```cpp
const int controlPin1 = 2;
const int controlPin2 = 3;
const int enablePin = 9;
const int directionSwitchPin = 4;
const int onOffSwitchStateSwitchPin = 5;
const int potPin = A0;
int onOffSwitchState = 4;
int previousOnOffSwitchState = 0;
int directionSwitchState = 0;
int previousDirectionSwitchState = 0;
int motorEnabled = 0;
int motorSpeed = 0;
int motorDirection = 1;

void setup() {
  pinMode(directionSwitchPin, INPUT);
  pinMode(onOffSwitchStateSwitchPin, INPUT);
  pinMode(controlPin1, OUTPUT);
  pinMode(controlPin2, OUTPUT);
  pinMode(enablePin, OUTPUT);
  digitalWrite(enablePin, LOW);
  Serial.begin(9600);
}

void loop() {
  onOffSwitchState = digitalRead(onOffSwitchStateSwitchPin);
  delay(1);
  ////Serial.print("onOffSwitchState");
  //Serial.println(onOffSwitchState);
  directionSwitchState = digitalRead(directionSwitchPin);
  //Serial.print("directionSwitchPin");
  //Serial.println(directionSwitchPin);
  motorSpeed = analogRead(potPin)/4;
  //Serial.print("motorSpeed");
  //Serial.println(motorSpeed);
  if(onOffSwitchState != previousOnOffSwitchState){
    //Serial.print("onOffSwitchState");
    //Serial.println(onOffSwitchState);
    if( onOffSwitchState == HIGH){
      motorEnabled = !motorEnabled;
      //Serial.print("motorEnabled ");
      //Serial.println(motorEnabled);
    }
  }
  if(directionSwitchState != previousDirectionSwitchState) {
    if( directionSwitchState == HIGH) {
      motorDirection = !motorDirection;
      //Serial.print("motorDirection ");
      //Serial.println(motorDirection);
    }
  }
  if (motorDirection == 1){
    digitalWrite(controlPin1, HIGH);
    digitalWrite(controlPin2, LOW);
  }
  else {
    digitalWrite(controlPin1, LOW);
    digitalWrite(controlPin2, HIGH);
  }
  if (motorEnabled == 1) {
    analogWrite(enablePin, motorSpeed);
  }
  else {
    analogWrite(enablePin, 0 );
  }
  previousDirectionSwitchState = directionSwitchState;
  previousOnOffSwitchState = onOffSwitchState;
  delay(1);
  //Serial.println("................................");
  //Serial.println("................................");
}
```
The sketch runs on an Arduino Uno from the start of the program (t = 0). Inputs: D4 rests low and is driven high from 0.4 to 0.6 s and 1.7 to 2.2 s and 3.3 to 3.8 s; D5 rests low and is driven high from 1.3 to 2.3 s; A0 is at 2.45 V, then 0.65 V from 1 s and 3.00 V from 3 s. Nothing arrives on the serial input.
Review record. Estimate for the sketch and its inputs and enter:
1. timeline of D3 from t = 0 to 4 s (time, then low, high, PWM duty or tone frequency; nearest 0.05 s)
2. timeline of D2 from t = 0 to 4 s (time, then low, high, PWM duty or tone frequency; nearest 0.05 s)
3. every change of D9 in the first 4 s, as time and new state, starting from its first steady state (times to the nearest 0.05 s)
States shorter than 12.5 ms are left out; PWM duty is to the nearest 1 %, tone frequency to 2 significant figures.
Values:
0 s low; 0.4 s high; 1.7 s low; 3.3 s high
0 s high; 0.4 s low; 1.7 s high; 3.3 s low
0 s low; 1.3 s PWM 13 %; 3 s PWM 60 %
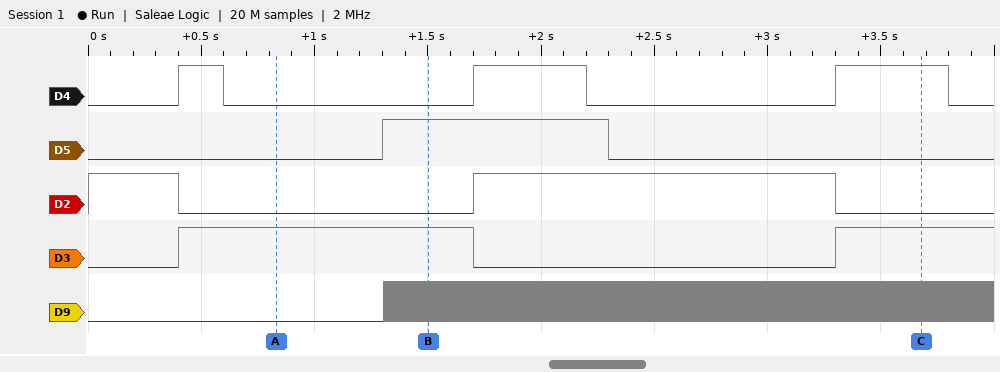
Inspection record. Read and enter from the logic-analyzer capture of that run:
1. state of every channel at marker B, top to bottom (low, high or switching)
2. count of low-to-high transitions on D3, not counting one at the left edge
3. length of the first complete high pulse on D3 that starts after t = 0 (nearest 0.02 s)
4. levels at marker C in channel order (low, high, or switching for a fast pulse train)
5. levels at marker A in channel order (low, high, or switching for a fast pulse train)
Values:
D4 low, D5 high, D2 low, D3 high, D9 switching
2
1.30 s
D4 high, D5 low, D2 low, D3 high, D9 switching
D4 low, D5 low, D2 low, D3 high, D9 low
